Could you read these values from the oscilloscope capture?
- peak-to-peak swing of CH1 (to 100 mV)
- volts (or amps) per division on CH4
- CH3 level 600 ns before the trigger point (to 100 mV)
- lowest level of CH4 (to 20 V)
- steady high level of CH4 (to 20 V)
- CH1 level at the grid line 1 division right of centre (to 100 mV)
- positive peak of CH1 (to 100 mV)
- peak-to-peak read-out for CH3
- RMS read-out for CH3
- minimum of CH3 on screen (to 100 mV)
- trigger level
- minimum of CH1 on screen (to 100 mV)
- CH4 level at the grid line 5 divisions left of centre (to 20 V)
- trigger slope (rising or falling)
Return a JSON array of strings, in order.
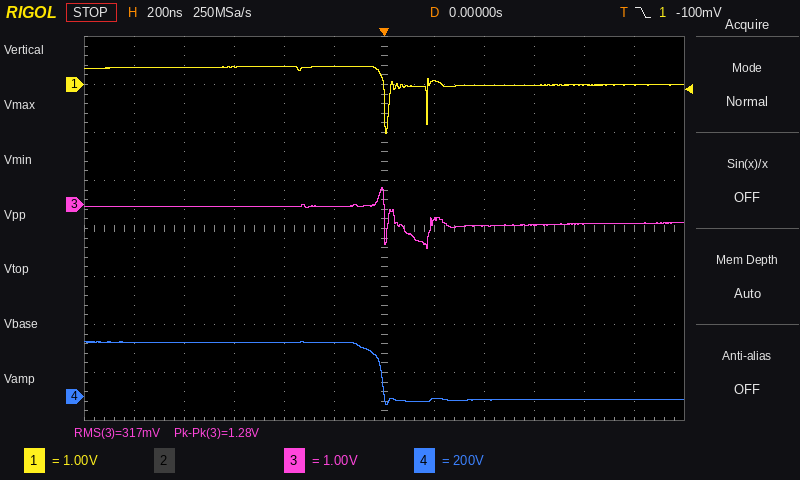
["1.4 V", "200 V", "0.0 V", "-40 V", "220 V", "100 mV", "400 mV", "1.28 V", "317 mV", "-900 mV", "-100 mV", "-1.0 V", "220 V", "falling"]
